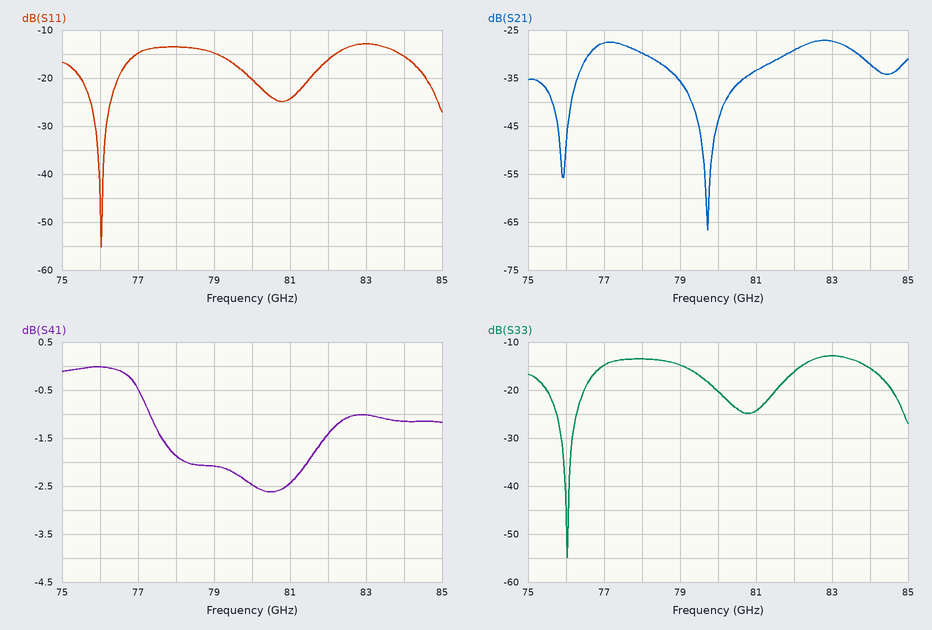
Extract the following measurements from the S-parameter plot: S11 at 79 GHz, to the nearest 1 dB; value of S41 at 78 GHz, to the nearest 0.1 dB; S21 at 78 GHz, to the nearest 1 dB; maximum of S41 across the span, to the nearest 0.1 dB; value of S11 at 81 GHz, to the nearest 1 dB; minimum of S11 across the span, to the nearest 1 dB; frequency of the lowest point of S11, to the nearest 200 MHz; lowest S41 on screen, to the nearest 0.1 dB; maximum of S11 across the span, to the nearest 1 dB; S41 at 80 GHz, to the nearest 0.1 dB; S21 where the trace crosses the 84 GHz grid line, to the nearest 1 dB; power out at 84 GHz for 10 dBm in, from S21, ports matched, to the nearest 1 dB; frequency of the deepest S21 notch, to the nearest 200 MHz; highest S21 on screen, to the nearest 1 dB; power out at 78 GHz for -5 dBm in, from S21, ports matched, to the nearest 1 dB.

-15 dB
-1.9 dB
-30 dB
0.0 dB
-24 dB
-55 dB
76.0 GHz
-2.6 dB
-13 dB
-2.5 dB
-32 dB
-22 dBm
79.8 GHz
-27 dB
-35 dBm
